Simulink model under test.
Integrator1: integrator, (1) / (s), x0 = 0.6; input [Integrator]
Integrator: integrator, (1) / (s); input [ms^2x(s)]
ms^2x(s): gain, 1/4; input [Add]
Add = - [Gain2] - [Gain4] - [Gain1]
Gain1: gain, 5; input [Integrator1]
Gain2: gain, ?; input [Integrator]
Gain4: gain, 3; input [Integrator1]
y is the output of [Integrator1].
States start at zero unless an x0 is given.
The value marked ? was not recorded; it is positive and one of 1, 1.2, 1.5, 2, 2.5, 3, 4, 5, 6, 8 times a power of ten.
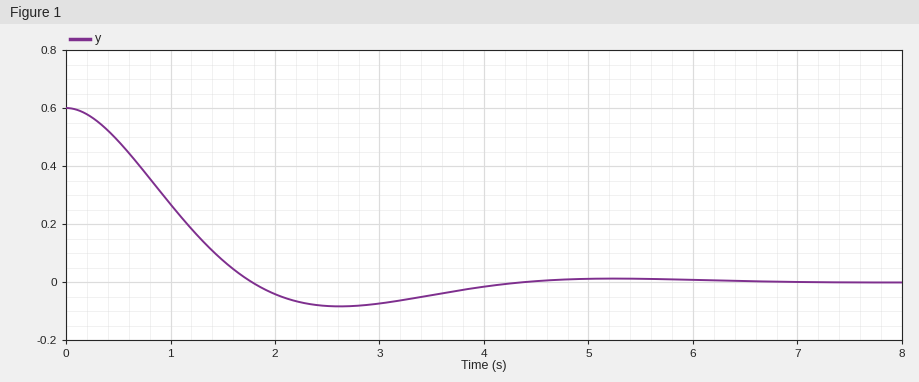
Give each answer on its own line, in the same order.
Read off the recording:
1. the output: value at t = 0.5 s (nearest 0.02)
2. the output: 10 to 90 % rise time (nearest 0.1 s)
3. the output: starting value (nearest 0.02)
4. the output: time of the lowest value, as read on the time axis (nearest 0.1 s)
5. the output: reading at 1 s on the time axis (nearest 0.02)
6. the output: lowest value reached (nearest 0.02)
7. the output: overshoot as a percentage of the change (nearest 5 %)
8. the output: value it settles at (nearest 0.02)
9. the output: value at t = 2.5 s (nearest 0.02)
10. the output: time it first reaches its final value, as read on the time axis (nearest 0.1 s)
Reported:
0.48
1.2 s
0.60
2.6 s
0.26
-0.08
15 %
0.00
-0.08
1.8 s
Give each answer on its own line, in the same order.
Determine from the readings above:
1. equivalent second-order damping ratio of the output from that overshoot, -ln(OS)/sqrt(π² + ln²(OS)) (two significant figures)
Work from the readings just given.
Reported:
0.52
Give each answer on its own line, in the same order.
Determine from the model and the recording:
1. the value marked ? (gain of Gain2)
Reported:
6
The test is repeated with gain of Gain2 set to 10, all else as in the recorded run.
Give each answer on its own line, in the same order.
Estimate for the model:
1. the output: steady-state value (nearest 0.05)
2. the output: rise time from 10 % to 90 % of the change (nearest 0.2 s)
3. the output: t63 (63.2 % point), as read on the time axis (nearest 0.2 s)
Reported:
0.00
2.0 s
1.4 s
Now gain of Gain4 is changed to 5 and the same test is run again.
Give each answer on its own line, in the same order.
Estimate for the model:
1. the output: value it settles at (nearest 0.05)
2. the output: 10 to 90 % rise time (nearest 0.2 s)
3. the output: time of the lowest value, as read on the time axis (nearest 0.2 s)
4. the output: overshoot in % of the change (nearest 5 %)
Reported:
0.00
1.0 s
2.2 s
20 %
